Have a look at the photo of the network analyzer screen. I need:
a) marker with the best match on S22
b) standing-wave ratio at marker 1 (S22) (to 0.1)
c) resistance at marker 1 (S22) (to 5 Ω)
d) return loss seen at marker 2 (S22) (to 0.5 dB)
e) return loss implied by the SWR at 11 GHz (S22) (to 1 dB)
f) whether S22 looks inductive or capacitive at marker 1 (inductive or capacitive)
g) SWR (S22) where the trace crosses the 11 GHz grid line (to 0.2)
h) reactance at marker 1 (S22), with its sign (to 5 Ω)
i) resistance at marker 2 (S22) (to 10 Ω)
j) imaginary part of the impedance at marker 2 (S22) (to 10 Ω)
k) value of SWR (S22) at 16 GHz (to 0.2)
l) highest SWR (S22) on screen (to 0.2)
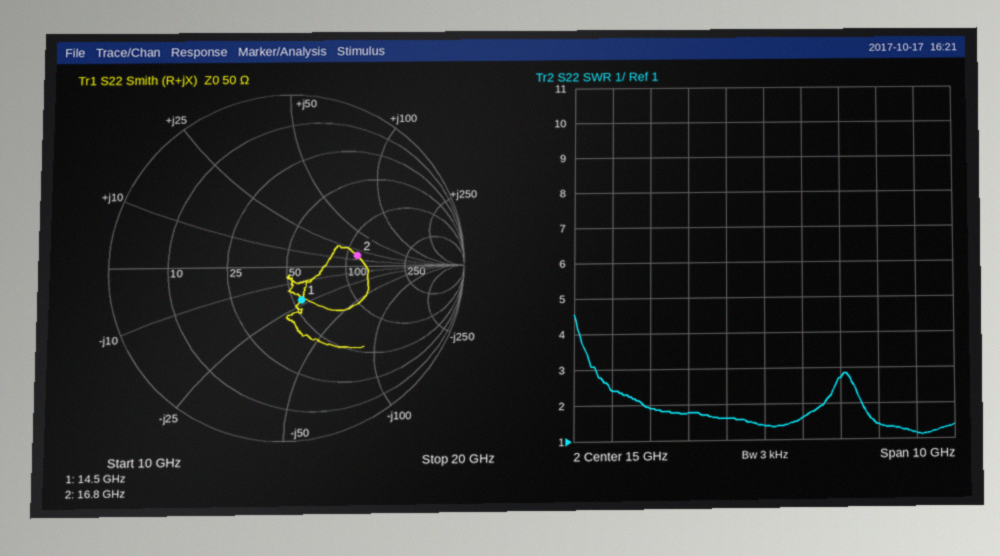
marker 1
1.5
55 Ω
8.0 dB
8 dB
capacitive
2.4
-20 Ω
110 Ω
+20 Ω
1.6
4.6
